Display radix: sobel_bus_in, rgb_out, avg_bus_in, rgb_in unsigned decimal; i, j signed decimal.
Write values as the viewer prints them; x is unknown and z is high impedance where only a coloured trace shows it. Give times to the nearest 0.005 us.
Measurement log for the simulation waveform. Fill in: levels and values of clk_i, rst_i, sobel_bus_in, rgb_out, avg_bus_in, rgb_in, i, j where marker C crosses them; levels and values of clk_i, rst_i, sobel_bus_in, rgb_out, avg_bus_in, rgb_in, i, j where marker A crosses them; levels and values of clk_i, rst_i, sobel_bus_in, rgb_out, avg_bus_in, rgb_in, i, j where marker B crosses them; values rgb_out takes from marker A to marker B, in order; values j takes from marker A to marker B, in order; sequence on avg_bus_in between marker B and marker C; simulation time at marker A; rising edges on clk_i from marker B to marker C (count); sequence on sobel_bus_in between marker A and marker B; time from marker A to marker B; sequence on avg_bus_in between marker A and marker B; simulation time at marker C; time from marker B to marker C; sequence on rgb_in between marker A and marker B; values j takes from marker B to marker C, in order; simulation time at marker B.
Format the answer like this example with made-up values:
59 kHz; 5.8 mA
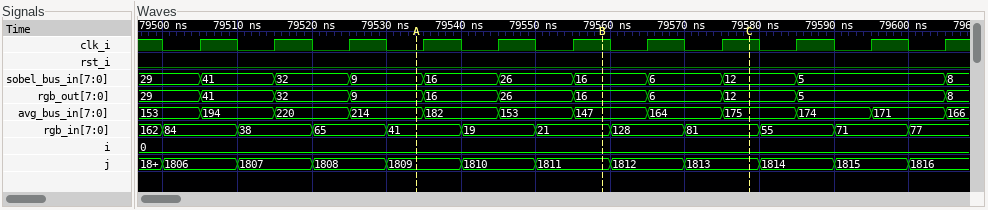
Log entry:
clk_i=1, rst_i=0, sobel_bus_in=12, rgb_out=12, avg_bus_in=175, rgb_in=81, i=0, j=1813; clk_i=0, rst_i=0, sobel_bus_in=9, rgb_out=9, avg_bus_in=214, rgb_in=41, i=0, j=1809; clk_i=1, rst_i=0, sobel_bus_in=16, rgb_out=16, avg_bus_in=147, rgb_in=21, i=0, j=1811; 9, 16, 26, 16; 1809, 1810, 1811; 147, 164, 175; 79.535 us; 2; 9, 16, 26, 16; 0.025 us; 214, 182, 153, 147; 79.58 us; 0.02 us; 41, 19, 21; 1811, 1812, 1813; 79.56 us
